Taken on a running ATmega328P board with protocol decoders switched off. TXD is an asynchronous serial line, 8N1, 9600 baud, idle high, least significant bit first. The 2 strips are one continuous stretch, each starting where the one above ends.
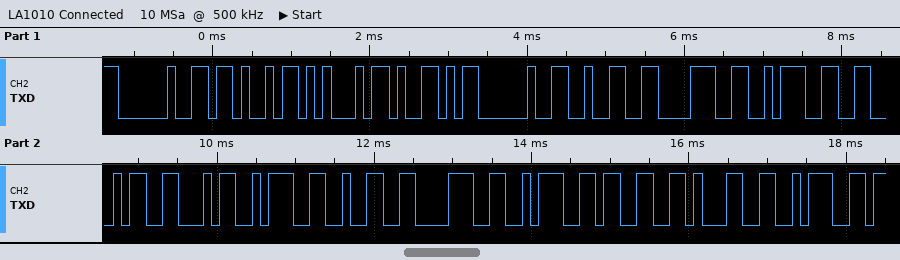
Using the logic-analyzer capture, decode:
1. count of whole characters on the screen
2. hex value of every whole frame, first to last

17
0x20 0x4B 0x45 0x59 0x20 0x32 0x38 0x3A 0x46 0x46 0x3A 0x32 0x38 0x3A 0x33 0x31 0x3A
